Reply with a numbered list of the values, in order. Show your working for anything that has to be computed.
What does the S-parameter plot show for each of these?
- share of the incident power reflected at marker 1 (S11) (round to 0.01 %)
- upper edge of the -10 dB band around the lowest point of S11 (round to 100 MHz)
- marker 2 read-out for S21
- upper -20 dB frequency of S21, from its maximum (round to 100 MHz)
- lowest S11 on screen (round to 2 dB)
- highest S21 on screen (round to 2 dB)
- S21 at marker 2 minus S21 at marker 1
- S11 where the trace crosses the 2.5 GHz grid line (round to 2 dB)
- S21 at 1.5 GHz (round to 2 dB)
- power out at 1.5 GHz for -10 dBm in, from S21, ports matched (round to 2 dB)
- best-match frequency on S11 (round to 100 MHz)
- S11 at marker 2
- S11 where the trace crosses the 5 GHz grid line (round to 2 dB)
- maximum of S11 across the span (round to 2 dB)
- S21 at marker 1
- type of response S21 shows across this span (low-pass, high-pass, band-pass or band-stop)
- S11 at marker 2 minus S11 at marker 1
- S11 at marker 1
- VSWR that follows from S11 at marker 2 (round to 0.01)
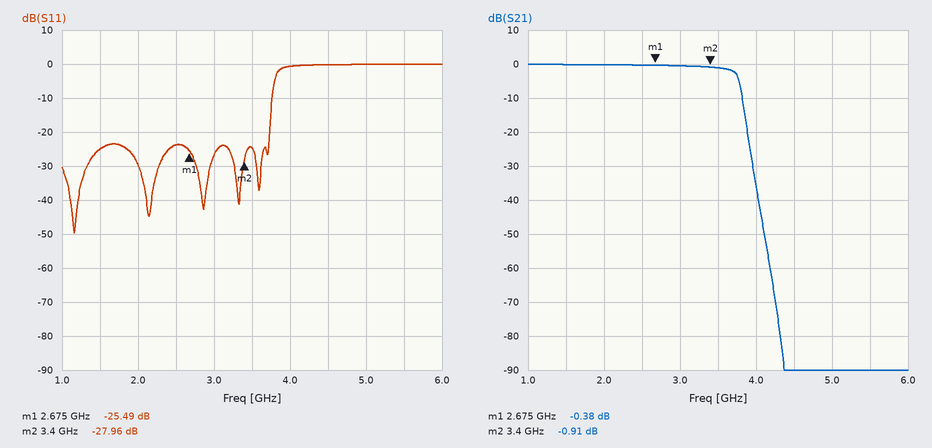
1. 10^(-25.49/10) ≈ 0.28 %
2. 3.8 GHz
3. -0.91 dB
4. 3.9 GHz
5. -50 dB
6. 0 dB
7. -0.91 − (-0.38) = -0.53 dB
8. -24 dB
9. 0 dB
10. -10 dBm + (0 dB) = -10 dBm
11. 1.2 GHz
12. -27.96 dB
13. 0 dB
14. 0 dB
15. -0.38 dB
16. low-pass
17. -27.96 − (-25.49) = -2.47 dB
18. -25.49 dB
19. (1 + 0.0400)/(1 − 0.0400) ≈ 1.08
